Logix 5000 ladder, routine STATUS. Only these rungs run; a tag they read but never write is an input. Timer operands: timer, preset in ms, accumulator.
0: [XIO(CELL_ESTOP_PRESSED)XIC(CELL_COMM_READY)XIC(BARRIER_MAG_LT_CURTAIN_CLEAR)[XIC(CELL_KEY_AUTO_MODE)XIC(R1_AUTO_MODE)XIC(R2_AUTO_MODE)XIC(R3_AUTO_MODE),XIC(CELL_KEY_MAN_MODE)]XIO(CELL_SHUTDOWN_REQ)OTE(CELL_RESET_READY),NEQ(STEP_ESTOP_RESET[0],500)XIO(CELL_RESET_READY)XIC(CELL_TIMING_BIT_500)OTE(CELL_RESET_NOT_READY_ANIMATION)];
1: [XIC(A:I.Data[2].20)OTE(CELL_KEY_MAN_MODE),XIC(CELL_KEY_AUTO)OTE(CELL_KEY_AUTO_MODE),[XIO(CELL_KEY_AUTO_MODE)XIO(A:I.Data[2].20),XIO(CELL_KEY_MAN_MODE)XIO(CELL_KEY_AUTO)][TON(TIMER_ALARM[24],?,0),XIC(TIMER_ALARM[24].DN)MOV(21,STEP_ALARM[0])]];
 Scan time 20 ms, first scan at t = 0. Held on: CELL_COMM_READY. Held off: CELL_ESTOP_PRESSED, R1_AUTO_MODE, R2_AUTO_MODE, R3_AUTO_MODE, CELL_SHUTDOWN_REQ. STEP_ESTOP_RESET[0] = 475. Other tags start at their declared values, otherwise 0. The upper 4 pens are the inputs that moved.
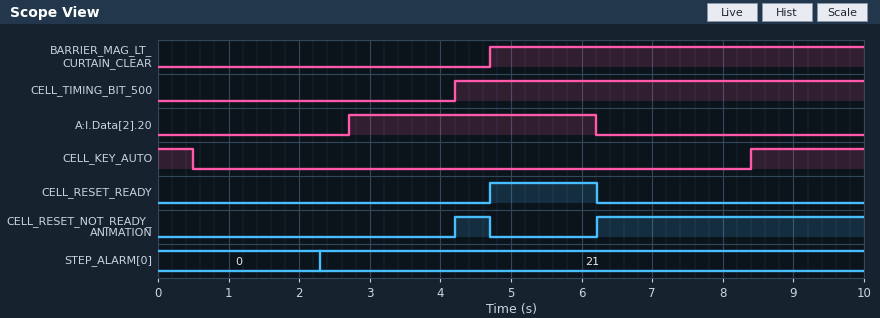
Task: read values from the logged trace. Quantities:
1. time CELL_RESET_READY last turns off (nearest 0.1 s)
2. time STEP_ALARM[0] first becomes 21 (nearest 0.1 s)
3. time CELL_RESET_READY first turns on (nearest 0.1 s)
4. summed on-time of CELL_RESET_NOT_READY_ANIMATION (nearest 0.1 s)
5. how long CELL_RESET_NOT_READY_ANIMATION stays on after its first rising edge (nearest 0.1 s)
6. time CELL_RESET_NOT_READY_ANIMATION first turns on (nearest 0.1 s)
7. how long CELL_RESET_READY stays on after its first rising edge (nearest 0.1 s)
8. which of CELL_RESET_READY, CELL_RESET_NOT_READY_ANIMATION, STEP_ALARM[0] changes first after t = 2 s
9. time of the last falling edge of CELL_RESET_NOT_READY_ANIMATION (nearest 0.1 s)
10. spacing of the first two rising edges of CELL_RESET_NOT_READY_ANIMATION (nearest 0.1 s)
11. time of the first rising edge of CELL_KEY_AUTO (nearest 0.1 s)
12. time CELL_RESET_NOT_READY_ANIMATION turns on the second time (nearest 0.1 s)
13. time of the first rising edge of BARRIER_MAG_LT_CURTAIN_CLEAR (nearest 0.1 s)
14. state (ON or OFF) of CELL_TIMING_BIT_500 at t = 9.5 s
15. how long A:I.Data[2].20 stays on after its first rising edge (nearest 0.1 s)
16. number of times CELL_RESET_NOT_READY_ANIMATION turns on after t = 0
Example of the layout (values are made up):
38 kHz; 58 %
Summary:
6.2 s; 2.3 s; 4.7 s; 4.3 s; 0.5 s; 4.2 s; 1.5 s; STEP_ALARM[0]; 4.7 s; 2.0 s; 8.4 s; 6.2 s; 4.7 s; ON; 3.5 s; 2
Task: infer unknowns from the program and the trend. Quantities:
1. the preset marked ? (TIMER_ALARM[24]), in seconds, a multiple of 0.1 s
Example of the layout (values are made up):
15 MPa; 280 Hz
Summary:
1.8 s
